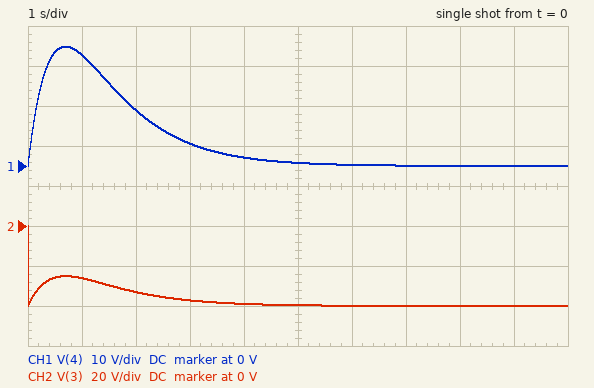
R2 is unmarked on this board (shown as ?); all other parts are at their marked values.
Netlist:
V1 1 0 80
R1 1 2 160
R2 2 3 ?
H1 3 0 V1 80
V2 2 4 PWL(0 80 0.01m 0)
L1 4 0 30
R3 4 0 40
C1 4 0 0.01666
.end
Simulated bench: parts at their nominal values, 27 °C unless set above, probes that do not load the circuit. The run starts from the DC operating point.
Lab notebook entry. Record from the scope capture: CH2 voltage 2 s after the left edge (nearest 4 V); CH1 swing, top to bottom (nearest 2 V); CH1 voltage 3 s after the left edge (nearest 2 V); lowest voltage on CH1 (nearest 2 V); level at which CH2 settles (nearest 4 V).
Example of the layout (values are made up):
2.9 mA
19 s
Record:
-32 V
30 V
6 V
0 V
-40 V
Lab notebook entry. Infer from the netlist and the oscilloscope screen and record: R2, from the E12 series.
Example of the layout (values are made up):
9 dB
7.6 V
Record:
27 Ω
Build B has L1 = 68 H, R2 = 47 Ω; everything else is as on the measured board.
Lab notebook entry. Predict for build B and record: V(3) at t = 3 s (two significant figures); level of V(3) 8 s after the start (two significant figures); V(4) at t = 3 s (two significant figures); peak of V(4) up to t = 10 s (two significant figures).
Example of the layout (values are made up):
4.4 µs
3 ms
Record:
-33 V
-39 V
14 V
26 V
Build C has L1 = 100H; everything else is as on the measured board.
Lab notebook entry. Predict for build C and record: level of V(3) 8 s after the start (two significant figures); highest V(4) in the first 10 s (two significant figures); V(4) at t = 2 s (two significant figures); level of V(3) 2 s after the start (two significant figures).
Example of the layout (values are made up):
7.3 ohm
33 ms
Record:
-36 V
35 V
30 V
-25 V
